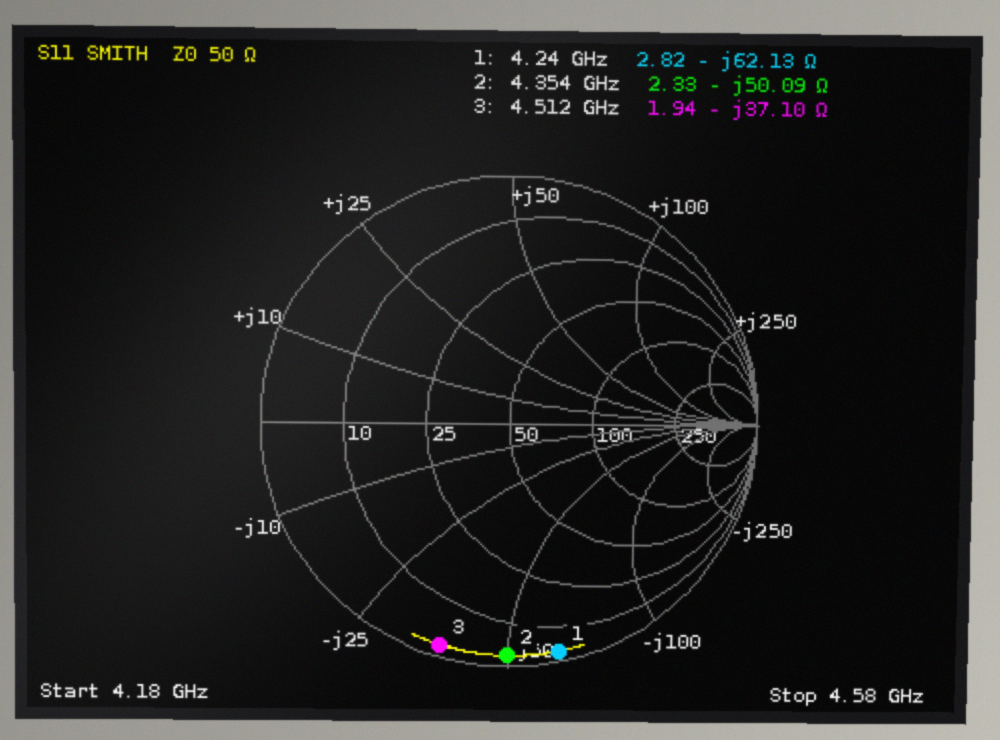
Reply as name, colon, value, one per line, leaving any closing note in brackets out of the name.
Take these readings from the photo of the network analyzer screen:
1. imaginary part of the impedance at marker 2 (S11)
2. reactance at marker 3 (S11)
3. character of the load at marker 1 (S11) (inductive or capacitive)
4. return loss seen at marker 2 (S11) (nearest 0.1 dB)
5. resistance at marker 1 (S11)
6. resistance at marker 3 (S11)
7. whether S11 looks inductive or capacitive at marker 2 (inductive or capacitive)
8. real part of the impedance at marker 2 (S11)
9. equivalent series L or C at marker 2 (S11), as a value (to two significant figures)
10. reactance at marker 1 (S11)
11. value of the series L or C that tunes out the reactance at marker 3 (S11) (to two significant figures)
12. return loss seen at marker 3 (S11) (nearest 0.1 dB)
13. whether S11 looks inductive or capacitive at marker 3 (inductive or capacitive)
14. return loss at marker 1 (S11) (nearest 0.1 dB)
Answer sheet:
imaginary part of the impedance at marker 2: -50.09 Ω
reactance at marker 3: -37.10 Ω
character of the load at marker 1 (S11): capacitive
return loss seen at marker 2 (S11): 0.4 dB
resistance at marker 1: 2.82 Ω
resistance at marker 3: 1.94 Ω
whether S11 looks inductive or capacitive at marker 2: capacitive
real part of the impedance at marker 2: 2.33 Ω
equivalent series L or C at marker 2 (S11), as a value: 730 fF
reactance at marker 1: -62.13 Ω
value of the series L or C that tunes out the reactance at marker 3 (S11): 1.3 nH
return loss seen at marker 3 (S11): 0.4 dB
whether S11 looks inductive or capacitive at marker 3: capacitive
return loss at marker 1 (S11): 0.4 dB
